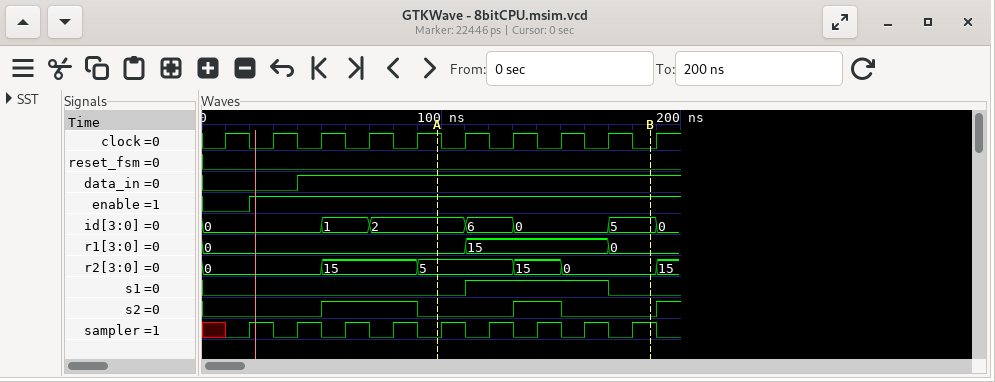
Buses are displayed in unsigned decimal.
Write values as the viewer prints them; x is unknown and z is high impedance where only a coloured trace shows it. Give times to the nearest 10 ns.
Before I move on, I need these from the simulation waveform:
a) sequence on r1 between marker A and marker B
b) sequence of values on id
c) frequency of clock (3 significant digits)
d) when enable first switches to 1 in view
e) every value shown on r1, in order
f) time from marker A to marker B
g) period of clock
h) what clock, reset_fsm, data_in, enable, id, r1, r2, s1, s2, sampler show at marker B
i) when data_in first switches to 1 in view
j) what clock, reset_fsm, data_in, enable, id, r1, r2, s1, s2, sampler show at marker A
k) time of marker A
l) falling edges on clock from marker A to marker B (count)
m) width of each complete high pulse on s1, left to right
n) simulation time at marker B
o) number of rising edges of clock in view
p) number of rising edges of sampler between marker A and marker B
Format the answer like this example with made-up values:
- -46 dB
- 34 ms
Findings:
- 0, 15, 0
- 0, 1, 2, 6, 0, 5, 0
- 50.0 MHz
- 20 ns
- 0, 15, 0
- 90 ns
- 20 ns
- clock=0, reset_fsm=0, data_in=1, enable=1, id=5, r1=0, r2=0, s1=0, s2=0, sampler=1
- 40 ns
- clock=1, reset_fsm=0, data_in=1, enable=1, id=2, r1=0, r2=5, s1=0, s2=0, sampler=0
- 100 ns
- 5
- 60 ns
- 190 ns
- 10
- 5
